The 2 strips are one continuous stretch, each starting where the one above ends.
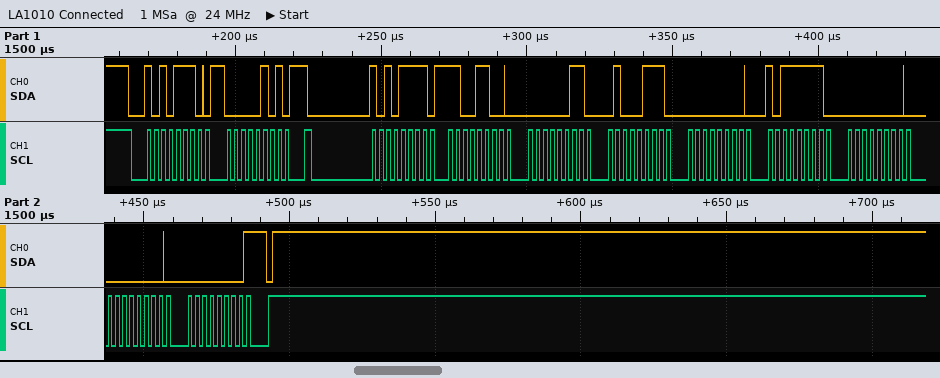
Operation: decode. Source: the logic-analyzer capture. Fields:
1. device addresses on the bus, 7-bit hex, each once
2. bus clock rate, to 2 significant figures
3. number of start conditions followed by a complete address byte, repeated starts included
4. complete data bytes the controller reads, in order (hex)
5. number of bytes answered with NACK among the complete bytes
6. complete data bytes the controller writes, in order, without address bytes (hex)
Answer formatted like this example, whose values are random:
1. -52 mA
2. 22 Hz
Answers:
1. 0x57
2. 400 kHz
3. 2
4. CC 03 47 00 BF 00 00 00
5. 1
6. 05
